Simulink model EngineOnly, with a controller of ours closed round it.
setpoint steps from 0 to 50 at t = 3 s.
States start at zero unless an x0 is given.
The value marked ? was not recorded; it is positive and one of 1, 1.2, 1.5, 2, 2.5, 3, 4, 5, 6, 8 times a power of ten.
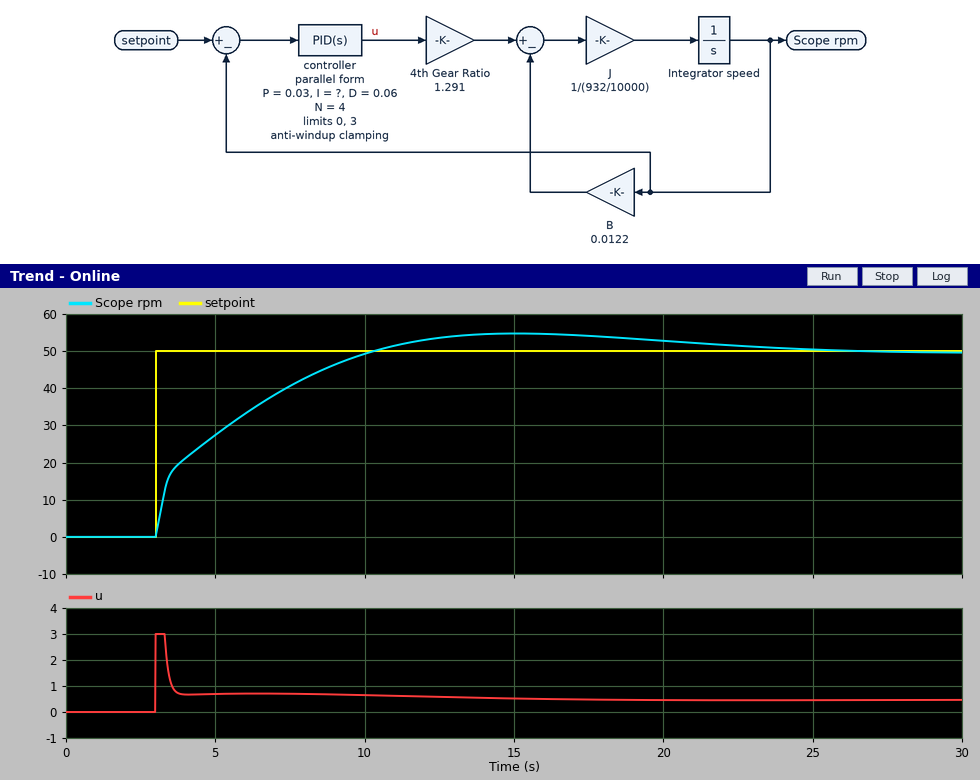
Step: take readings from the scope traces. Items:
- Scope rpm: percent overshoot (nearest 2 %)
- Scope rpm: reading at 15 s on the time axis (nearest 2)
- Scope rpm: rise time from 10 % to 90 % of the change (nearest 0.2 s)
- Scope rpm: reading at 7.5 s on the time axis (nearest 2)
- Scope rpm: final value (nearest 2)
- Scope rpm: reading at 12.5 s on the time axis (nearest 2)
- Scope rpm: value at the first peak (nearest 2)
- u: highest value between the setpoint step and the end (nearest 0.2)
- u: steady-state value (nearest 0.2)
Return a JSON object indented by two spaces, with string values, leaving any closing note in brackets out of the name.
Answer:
{
  "Scope rpm: percent overshoot": "10 %",
  "Scope rpm: reading at 15 s on the time axis": "54",
  "Scope rpm: rise time from 10 % to 90 % of the change": "5.4 s",
  "Scope rpm: reading at 7.5 s on the time axis": "40",
  "Scope rpm: final value": "50",
  "Scope rpm: reading at 12.5 s on the time axis": "54",
  "Scope rpm: value at the first peak": "54",
  "u: highest value between the setpoint step and the end": "3.0",
  "u: steady-state value": "0.4"
}
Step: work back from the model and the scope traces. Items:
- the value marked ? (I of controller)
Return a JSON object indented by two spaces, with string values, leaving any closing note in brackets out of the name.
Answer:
{
  "the value marked ?": "0.008"
}
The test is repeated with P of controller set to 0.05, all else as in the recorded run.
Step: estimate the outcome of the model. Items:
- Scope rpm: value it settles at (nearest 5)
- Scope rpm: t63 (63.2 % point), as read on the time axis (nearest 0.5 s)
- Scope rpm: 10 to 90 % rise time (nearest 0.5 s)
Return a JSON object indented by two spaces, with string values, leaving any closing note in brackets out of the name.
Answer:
{
  "Scope rpm: value it settles at": "50",
  "Scope rpm: t63 (63.2 % point), as read on the time axis": "5.0 s",
  "Scope rpm: 10 to 90 % rise time": "4.5 s"
}
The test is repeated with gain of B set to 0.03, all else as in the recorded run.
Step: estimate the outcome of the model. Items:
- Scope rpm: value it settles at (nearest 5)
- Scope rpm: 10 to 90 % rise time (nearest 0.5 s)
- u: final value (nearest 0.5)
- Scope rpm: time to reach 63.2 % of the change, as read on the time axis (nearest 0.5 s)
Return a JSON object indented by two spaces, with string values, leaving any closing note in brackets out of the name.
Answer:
{
  "Scope rpm: value it settles at": "50",
  "Scope rpm: 10 to 90 % rise time": "8.5 s",
  "u: final value": "1.0",
  "Scope rpm: time to reach 63.2 % of the change, as read on the time axis": "6.5 s"
}
